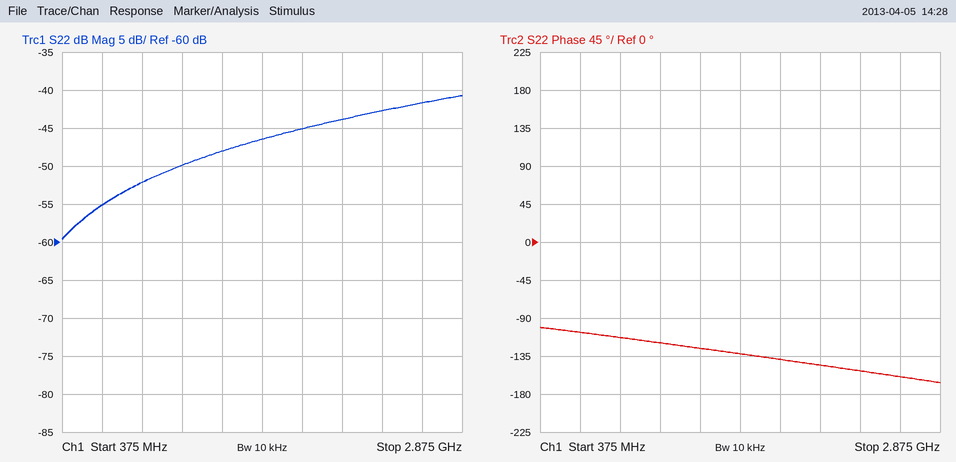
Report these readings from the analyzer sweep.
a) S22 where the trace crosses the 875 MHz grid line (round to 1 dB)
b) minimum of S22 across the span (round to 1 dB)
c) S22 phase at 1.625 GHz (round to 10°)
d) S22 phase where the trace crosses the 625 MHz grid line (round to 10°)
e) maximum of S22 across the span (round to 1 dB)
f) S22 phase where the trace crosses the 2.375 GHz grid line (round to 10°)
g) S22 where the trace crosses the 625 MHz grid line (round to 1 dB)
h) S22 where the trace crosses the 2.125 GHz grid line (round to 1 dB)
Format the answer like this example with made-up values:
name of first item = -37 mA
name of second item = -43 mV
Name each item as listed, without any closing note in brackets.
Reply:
S22 where the trace crosses the 875 MHz grid line = -52 dB
minimum of S22 across the span = -60 dB
S22 phase at 1.625 GHz = -130°
S22 phase where the trace crosses the 625 MHz grid line = -110°
maximum of S22 across the span = -41 dB
S22 phase where the trace crosses the 2.375 GHz grid line = -150°
S22 where the trace crosses the 625 MHz grid line = -55 dB
S22 where the trace crosses the 2.125 GHz grid line = -44 dB
